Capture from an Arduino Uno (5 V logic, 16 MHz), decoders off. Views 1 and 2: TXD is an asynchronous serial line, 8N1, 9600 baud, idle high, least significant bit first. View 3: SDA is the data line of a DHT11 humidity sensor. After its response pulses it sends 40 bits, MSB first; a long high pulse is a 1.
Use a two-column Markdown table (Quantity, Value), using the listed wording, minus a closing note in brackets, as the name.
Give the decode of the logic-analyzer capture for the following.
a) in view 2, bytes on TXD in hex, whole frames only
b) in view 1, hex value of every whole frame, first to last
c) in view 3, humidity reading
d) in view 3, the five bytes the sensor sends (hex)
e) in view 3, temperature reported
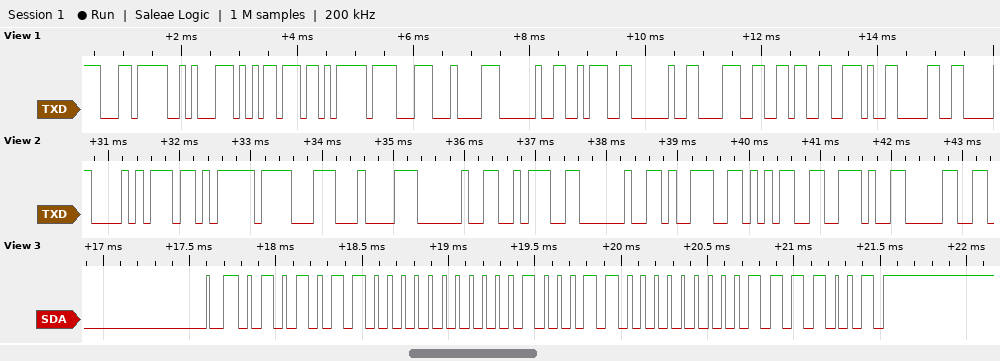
| Quantity | Value |
|---|---|
| in view 2, bytes on TXD in hex, whole frames only | A8 EB 8F 84 20 3A 20 39 35 2E 30 |
| in view 1, hex value of every whole frame, first to last | EC 8A B5 EB 8F 84 20 3A 20 38 36 2E 30 |
| in view 3, humidity reading | 86 % |
| in view 3, the five bytes the sensor sends | 56 00 23 00 79 |
| in view 3, temperature reported | 35.0 °C |
